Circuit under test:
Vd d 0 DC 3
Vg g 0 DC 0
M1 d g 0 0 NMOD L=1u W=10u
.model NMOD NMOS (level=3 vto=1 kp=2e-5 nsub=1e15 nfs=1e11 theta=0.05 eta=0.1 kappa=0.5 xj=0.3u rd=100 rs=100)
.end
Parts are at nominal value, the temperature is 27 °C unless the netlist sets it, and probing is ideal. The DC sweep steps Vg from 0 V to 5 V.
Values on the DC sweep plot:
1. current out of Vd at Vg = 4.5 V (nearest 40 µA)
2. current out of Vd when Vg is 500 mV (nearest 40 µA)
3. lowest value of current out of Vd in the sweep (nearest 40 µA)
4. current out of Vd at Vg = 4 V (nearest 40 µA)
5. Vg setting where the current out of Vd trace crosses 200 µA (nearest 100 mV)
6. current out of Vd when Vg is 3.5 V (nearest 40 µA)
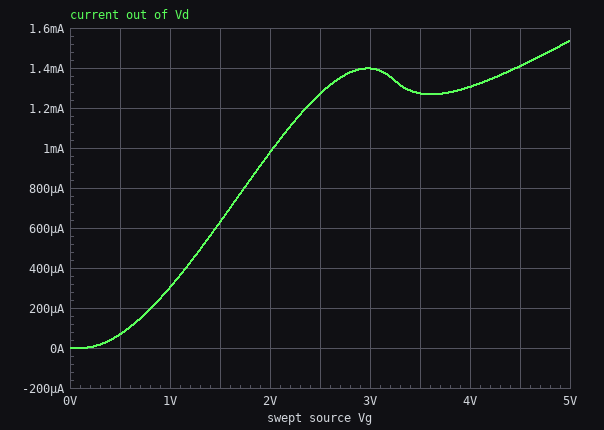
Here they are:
1.40 mA
80 µA
0 A
1.32 mA
800 mV
1.28 mA
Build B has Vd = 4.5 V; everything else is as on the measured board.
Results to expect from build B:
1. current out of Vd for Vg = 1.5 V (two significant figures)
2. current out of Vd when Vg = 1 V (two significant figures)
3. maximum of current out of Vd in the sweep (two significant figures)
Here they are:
1.2 mA
680 µA
3.2 mA
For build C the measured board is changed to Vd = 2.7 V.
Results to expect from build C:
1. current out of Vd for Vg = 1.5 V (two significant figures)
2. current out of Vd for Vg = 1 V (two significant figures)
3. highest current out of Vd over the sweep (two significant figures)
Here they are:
540 µA
250 µA
1.4 mA
